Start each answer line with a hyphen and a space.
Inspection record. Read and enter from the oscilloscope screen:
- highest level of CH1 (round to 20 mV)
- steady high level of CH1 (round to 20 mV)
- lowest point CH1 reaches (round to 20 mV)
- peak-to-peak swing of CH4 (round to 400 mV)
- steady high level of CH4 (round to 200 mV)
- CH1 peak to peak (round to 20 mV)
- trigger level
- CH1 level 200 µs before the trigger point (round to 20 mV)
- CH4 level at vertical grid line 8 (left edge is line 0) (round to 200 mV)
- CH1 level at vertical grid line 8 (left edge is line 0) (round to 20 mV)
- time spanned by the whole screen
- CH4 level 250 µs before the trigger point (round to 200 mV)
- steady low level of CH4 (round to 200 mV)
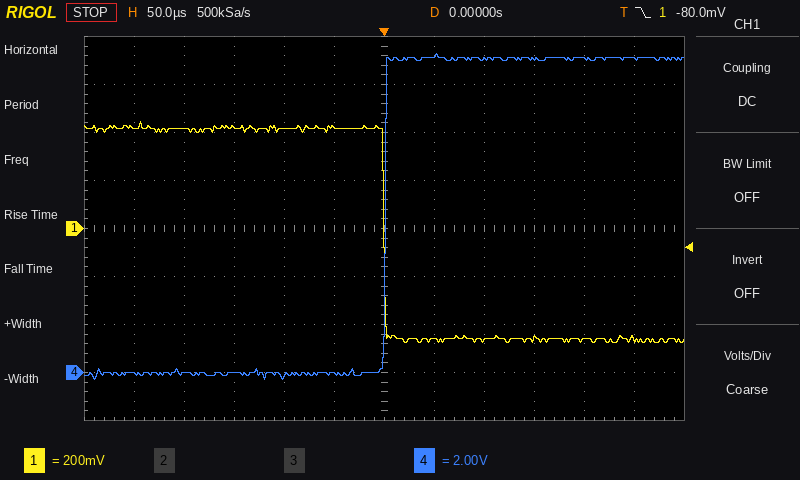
- 440 mV
- 420 mV
- -480 mV
- 13.6 V
- 13.2 V
- 920 mV
- -80.0 mV
- 420 mV
- 13.0 V
- -460 mV
- 600 µs
- 0.0 V
- 0.0 V
